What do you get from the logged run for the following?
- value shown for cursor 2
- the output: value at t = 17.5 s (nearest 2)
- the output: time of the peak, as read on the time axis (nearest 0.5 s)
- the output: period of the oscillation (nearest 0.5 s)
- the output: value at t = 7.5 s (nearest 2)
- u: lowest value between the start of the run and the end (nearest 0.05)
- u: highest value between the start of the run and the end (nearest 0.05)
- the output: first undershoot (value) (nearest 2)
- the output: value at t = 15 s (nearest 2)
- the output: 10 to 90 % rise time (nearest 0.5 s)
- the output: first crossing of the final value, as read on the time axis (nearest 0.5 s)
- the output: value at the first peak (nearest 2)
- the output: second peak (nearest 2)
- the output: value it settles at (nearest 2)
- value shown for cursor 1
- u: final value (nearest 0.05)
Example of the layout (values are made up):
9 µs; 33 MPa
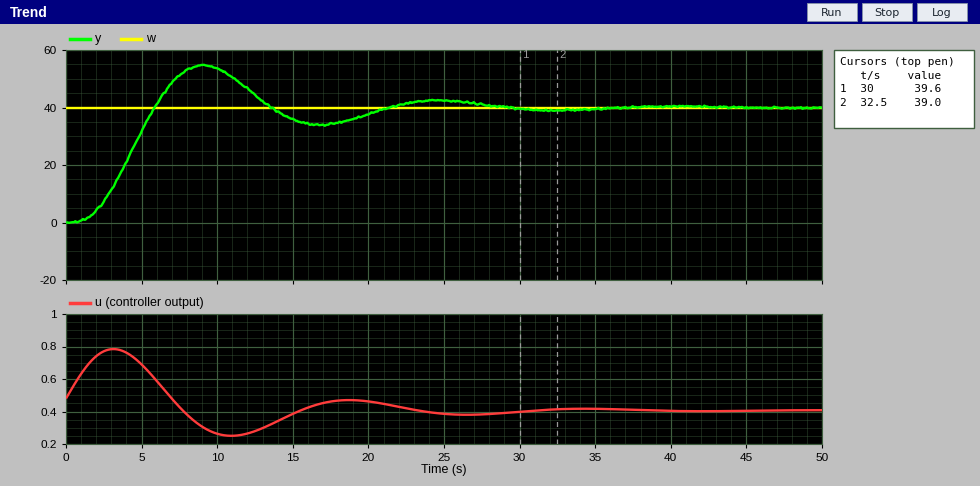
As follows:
39.0; 34; 9.0 s; 15.5 s; 52; 0.25; 0.80; 34; 36; 3.5 s; 6.0 s; 54; 42; 40; 39.6; 0.40
